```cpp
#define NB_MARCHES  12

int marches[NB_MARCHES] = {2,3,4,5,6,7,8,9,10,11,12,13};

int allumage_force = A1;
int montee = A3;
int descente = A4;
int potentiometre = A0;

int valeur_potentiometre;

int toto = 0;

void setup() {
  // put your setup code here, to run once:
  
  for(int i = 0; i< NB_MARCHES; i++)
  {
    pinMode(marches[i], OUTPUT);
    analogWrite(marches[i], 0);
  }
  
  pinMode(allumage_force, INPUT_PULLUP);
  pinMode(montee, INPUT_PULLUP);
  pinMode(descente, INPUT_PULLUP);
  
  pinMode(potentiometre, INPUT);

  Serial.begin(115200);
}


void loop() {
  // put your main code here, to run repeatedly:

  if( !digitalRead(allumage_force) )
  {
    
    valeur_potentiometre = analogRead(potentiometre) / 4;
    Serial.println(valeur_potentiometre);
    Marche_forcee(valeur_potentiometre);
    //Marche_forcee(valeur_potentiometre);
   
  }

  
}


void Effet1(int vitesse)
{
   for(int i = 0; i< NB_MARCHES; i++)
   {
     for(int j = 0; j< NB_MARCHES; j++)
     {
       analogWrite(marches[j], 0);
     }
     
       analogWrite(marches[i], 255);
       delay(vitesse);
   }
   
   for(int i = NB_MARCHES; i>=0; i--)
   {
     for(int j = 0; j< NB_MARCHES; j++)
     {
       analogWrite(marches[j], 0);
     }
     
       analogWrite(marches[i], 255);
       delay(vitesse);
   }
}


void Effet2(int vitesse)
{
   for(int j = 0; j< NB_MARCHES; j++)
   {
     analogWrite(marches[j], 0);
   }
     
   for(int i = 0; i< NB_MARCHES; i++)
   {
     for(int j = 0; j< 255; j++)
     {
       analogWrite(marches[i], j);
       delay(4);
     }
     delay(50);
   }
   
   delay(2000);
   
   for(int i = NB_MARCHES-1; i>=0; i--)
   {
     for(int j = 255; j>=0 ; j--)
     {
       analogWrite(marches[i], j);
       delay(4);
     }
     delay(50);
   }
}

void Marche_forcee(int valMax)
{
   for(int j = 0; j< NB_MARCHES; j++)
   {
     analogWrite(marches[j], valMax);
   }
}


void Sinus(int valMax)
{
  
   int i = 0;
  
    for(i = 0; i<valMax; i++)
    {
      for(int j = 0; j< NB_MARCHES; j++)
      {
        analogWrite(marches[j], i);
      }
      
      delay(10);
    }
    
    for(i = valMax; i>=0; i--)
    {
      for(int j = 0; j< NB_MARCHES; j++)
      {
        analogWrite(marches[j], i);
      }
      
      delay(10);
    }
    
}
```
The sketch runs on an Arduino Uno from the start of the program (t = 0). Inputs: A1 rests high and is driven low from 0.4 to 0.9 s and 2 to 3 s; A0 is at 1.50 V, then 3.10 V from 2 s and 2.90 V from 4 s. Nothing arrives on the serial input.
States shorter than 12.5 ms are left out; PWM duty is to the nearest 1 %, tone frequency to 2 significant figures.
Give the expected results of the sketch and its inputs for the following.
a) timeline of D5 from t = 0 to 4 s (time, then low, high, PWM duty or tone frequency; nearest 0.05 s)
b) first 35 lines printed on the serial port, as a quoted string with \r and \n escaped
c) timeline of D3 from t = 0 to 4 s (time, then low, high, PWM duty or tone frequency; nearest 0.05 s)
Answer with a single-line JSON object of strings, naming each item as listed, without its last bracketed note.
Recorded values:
{"timeline of D5 from t = 0 to 4 s": "0 s low; 0.4 s PWM 30 %; 2 s PWM 62 %", "first 35 lines printed on the serial port, as a quoted string with \\r and \\n escaped": "\"76\\r\\n76\\r\\n76\\r\\n76\\r\\n76\\r\\n76\\r\\n76\\r\\n76\\r\\n76\\r\\n76\\r\\n76\\r\\n76\\r\\n76\\r\\n76\\r\\n76\\r\\n76\\r\\n76\\r\\n76\\r\\n76\\r\\n76\\r\\n76\\r\\n76\\r\\n76\\r\\n76\\r\\n76\\r\\n76\\r\\n76\\r\\n76\\r\\n76\\r\\n76\\r\\n76\\r\\n76\\r\\n76\\r\\n76\\r\\n76\\r\\n\"", "timeline of D3 from t = 0 to 4 s": "0 s low; 0.4 s PWM 30 %; 2 s PWM 62 %"}
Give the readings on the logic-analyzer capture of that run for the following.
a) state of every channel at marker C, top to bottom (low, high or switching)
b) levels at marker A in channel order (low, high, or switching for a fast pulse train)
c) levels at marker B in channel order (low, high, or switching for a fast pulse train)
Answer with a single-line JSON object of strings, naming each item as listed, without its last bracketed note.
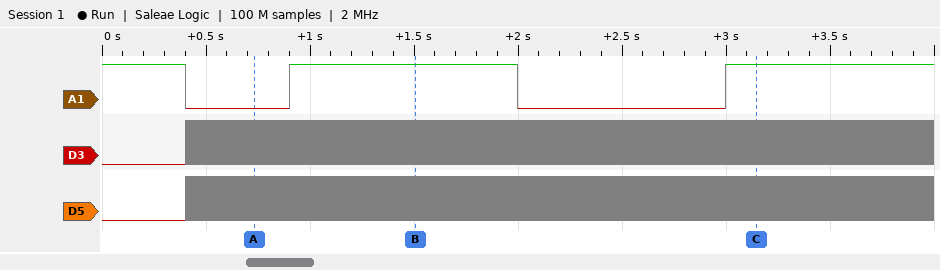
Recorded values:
{"state of every channel at marker C, top to bottom": "A1 high, D3 switching, D5 switching", "levels at marker A in channel order": "A1 low, D3 switching, D5 switching", "levels at marker B in channel order": "A1 high, D3 switching, D5 switching"}
